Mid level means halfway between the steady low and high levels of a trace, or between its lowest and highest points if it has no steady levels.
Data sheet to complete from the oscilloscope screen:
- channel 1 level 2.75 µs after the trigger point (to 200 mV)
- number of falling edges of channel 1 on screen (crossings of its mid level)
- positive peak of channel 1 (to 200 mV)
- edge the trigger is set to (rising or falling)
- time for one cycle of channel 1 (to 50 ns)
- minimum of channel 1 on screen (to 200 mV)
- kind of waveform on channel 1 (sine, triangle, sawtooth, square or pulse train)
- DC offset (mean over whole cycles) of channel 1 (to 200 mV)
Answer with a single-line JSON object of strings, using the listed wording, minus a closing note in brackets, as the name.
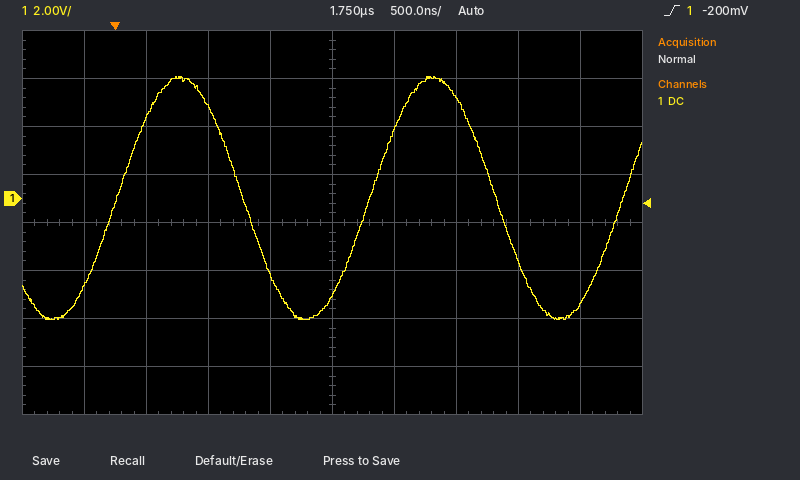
{"channel 1 level 2.75 µs after the trigger point": "4.2 V", "number of falling edges of channel 1 on screen": "2", "positive peak of channel 1": "5.0 V", "edge the trigger is set to": "rising", "time for one cycle of channel 1": "2.05 µs", "minimum of channel 1 on screen": "-5.0 V", "kind of waveform on channel 1": "sine", "DC offset (mean over whole cycles) of channel 1": "0.0 V"}
